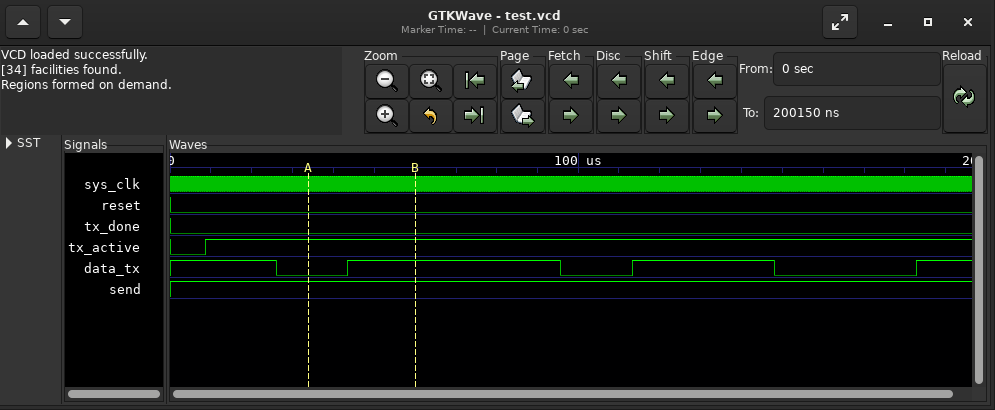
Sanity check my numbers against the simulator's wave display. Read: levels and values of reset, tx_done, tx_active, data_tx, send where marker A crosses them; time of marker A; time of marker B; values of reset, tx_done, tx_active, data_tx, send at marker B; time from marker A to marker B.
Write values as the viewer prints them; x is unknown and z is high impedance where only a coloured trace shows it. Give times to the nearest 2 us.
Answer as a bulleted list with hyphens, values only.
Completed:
- reset=0, tx_done=0, tx_active=1, data_tx=0, send=1
- 34 us
- 60 us
- reset=0, tx_done=0, tx_active=1, data_tx=1, send=1
- 26 us
